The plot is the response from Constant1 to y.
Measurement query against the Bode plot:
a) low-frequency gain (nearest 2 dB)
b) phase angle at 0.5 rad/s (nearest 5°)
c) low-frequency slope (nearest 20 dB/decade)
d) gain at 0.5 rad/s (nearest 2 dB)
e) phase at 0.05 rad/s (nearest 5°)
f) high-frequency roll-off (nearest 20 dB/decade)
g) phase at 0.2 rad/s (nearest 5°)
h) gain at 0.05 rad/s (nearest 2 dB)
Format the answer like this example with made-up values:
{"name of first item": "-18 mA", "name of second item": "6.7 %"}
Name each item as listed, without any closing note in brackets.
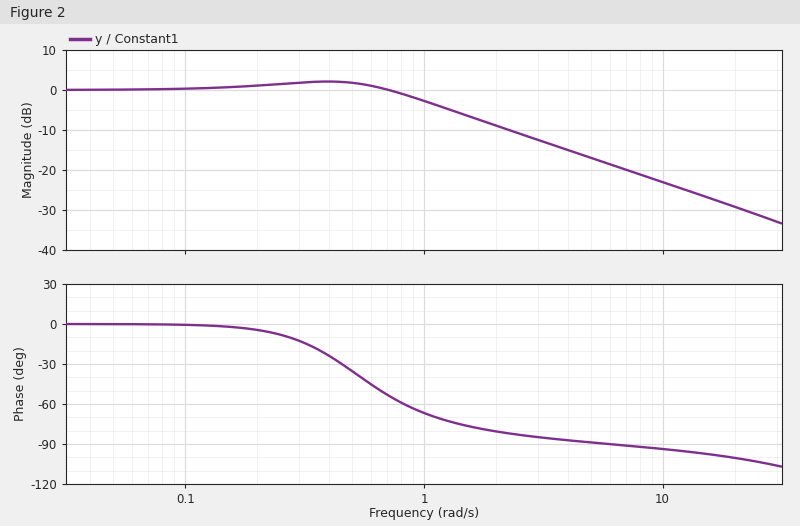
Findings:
{"low-frequency gain": "0 dB", "phase angle at 0.5 rad/s": "-35°", "low-frequency slope": "0 dB/decade", "gain at 0.5 rad/s": "2 dB", "phase at 0.05 rad/s": "0°", "high-frequency roll-off": "-20 dB/decade", "phase at 0.2 rad/s": "-5°", "gain at 0.05 rad/s": "0 dB"}
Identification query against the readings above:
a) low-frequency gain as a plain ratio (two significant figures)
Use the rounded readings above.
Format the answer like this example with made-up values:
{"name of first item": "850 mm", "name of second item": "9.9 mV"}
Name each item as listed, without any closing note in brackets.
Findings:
{"low-frequency gain as a plain ratio": "1.0"}
